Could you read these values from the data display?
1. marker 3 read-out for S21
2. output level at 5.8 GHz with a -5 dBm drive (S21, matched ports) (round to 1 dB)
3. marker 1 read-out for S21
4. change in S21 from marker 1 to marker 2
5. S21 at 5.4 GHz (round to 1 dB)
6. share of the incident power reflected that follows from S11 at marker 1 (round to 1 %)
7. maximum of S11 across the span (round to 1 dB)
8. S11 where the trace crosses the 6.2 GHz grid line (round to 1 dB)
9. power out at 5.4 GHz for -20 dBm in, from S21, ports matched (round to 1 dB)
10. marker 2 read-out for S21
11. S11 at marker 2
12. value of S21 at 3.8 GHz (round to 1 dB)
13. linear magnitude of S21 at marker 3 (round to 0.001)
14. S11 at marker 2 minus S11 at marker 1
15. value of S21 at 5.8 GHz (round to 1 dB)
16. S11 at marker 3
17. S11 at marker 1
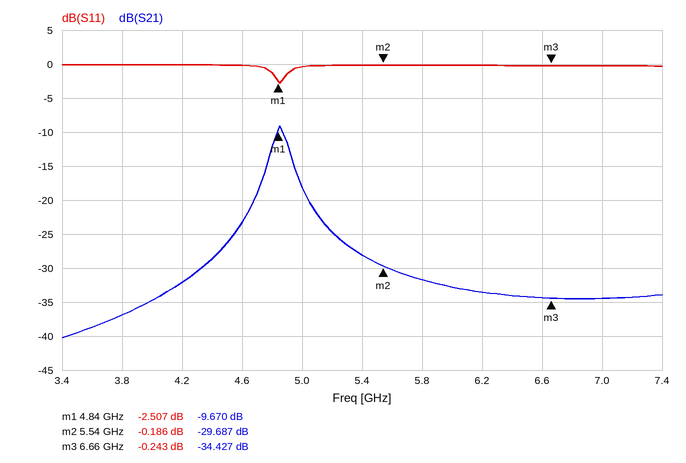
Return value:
-34.427 dB
-37 dBm
-9.670 dB
-20.017 dB
-28 dB
56 %
0 dB
0 dB
-48 dBm
-29.687 dB
-0.186 dB
-37 dB
0.019
2.321 dB
-32 dB
-0.243 dB
-2.507 dB
